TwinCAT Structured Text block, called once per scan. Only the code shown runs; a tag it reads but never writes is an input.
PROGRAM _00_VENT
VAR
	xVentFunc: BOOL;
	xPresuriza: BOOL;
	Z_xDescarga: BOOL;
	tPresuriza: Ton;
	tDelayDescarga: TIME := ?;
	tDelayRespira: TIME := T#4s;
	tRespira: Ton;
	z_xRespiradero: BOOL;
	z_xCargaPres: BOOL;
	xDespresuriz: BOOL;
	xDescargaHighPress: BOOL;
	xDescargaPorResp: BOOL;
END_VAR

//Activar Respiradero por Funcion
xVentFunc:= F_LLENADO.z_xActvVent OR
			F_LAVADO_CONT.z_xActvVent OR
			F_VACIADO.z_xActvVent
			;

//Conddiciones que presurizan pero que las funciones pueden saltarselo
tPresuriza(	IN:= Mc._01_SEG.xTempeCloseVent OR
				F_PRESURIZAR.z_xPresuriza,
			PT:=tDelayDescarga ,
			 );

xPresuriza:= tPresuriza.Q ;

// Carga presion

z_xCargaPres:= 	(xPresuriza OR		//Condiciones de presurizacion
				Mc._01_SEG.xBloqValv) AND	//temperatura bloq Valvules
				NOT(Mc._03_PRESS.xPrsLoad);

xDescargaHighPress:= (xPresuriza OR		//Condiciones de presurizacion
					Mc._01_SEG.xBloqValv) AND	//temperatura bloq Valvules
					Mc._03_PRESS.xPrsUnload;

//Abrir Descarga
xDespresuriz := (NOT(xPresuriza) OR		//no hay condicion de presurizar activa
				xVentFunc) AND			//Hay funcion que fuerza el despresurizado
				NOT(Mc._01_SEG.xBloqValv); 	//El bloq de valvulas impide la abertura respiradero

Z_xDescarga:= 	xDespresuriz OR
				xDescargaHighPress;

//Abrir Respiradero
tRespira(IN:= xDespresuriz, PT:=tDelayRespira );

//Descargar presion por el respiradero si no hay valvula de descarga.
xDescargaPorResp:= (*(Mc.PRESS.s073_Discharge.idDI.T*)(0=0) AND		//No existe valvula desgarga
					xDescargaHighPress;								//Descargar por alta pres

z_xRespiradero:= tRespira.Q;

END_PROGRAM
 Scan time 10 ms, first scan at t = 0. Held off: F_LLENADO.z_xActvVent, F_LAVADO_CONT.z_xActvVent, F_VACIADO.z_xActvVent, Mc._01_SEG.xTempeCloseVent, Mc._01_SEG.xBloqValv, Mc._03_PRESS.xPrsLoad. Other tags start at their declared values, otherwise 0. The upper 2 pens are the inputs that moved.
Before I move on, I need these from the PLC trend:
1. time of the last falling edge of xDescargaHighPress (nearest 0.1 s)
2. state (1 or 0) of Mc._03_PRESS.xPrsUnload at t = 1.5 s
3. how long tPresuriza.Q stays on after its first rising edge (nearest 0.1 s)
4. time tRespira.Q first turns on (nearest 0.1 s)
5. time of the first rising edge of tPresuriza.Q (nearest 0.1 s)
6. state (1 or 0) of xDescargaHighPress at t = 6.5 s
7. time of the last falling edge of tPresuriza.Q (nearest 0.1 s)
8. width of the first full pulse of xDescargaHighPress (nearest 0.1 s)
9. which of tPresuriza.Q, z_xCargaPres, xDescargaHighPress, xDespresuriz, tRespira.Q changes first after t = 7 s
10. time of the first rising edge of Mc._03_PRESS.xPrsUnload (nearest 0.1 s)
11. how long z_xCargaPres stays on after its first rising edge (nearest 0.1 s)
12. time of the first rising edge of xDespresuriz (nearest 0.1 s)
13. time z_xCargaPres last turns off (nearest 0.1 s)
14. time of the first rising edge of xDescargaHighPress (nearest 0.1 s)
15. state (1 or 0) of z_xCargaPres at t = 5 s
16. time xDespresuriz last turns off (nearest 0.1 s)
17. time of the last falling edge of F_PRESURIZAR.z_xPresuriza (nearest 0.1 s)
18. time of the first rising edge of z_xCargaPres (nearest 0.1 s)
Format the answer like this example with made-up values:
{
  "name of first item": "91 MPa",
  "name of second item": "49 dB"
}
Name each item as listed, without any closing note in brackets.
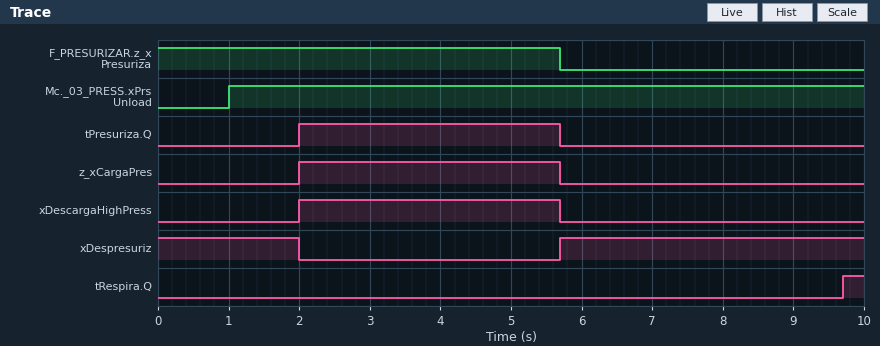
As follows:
{
  "time of the last falling edge of xDescargaHighPress": "5.7 s",
  "state (1 or 0) of Mc._03_PRESS.xPrsUnload at t = 1.5 s": "1",
  "how long tPresuriza.Q stays on after its first rising edge": "3.7 s",
  "time tRespira.Q first turns on": "9.7 s",
  "time of the first rising edge of tPresuriza.Q": "2.0 s",
  "state (1 or 0) of xDescargaHighPress at t = 6.5 s": "0",
  "time of the last falling edge of tPresuriza.Q": "5.7 s",
  "width of the first full pulse of xDescargaHighPress": "3.7 s",
  "which of tPresuriza.Q, z_xCargaPres, xDescargaHighPress, xDespresuriz, tRespira.Q changes first after t = 7 s": "tRespira.Q",
  "time of the first rising edge of Mc._03_PRESS.xPrsUnload": "1.0 s",
  "how long z_xCargaPres stays on after its first rising edge": "3.7 s",
  "time of the first rising edge of xDespresuriz": "5.7 s",
  "time z_xCargaPres last turns off": "5.7 s",
  "time of the first rising edge of xDescargaHighPress": "2.0 s",
  "state (1 or 0) of z_xCargaPres at t = 5 s": "1",
  "time xDespresuriz last turns off": "2.0 s",
  "time of the last falling edge of F_PRESURIZAR.z_xPresuriza": "5.7 s",
  "time of the first rising edge of z_xCargaPres": "2.0 s"
}
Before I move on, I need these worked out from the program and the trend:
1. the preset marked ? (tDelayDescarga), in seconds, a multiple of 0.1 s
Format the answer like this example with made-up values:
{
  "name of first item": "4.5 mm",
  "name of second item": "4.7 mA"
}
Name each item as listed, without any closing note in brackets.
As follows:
{
  "the preset marked ? (tDelayDescarga), in seconds, a multiple of 0.1 s": "2.0 s"
}
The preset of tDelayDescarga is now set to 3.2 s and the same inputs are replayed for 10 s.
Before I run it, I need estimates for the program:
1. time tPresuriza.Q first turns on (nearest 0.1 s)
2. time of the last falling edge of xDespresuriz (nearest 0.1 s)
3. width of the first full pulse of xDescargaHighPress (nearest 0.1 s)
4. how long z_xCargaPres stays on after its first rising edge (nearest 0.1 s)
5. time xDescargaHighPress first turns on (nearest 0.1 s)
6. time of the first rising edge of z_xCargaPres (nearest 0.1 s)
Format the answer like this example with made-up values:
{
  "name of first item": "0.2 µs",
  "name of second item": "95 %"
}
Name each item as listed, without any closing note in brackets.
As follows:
{
  "time tPresuriza.Q first turns on": "3.2 s",
  "time of the last falling edge of xDespresuriz": "3.2 s",
  "width of the first full pulse of xDescargaHighPress": "2.5 s",
  "how long z_xCargaPres stays on after its first rising edge": "2.5 s",
  "time xDescargaHighPress first turns on": "3.2 s",
  "time of the first rising edge of z_xCargaPres": "3.2 s"
}
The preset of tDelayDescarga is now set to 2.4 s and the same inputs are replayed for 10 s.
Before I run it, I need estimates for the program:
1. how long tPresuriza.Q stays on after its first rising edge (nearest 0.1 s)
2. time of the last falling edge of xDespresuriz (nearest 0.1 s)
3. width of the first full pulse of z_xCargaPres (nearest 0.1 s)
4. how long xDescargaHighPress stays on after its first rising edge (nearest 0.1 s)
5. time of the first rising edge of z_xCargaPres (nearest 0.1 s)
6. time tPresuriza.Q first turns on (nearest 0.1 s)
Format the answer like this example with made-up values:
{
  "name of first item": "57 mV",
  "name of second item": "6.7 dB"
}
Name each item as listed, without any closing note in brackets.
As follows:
{
  "how long tPresuriza.Q stays on after its first rising edge": "3.3 s",
  "time of the last falling edge of xDespresuriz": "2.4 s",
  "width of the first full pulse of z_xCargaPres": "3.3 s",
  "how long xDescargaHighPress stays on after its first rising edge": "3.3 s",
  "time of the first rising edge of z_xCargaPres": "2.4 s",
  "time tPresuriza.Q first turns on": "2.4 s"
}
